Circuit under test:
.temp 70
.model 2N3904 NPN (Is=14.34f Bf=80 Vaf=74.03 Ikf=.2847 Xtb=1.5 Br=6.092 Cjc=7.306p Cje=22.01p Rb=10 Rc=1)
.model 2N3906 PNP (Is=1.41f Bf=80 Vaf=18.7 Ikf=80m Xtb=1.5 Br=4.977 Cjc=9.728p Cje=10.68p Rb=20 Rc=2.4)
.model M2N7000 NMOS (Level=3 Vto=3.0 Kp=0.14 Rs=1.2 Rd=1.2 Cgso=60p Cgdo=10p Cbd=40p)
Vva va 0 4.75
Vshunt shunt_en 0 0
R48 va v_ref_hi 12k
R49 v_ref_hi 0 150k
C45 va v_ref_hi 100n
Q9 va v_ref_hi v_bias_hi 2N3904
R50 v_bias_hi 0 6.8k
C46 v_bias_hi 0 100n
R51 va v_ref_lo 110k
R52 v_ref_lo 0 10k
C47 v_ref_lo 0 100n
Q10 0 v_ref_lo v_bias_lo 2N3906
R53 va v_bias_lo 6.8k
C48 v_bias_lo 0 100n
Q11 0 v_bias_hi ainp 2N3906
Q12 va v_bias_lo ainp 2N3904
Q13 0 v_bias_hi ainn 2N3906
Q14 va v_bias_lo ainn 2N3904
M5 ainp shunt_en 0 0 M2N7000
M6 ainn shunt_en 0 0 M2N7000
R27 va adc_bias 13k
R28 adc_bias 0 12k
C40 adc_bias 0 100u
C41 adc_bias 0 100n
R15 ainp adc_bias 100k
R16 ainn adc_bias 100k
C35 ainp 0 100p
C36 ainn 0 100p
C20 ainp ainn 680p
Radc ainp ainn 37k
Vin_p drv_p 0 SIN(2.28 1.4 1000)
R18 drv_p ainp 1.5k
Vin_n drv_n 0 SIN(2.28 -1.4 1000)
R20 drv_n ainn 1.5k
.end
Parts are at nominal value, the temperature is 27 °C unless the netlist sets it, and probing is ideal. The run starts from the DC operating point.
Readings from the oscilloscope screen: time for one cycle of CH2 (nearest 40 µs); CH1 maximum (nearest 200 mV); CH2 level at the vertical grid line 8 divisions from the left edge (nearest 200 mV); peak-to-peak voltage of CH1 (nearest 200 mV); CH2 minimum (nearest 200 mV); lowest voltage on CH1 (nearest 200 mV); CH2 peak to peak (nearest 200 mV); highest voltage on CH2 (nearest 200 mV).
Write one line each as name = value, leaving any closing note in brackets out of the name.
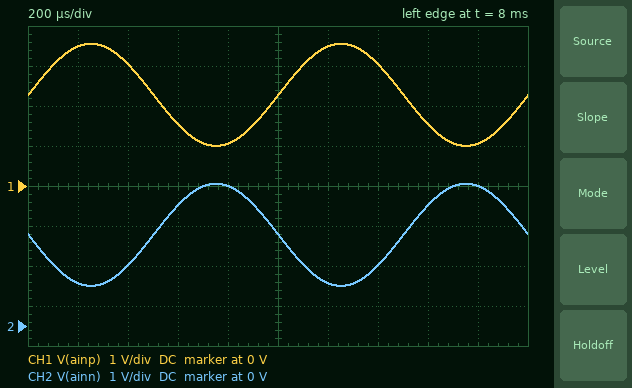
time for one cycle of CH2 = 1.00 ms
CH1 maximum = 3.6 V
CH2 level at the vertical grid line 8 divisions from the left edge = 3.0 V
peak-to-peak voltage of CH1 = 2.6 V
CH2 minimum = 1.0 V
lowest voltage on CH1 = 1.0 V
CH2 peak to peak = 2.6 V
highest voltage on CH2 = 3.6 V
